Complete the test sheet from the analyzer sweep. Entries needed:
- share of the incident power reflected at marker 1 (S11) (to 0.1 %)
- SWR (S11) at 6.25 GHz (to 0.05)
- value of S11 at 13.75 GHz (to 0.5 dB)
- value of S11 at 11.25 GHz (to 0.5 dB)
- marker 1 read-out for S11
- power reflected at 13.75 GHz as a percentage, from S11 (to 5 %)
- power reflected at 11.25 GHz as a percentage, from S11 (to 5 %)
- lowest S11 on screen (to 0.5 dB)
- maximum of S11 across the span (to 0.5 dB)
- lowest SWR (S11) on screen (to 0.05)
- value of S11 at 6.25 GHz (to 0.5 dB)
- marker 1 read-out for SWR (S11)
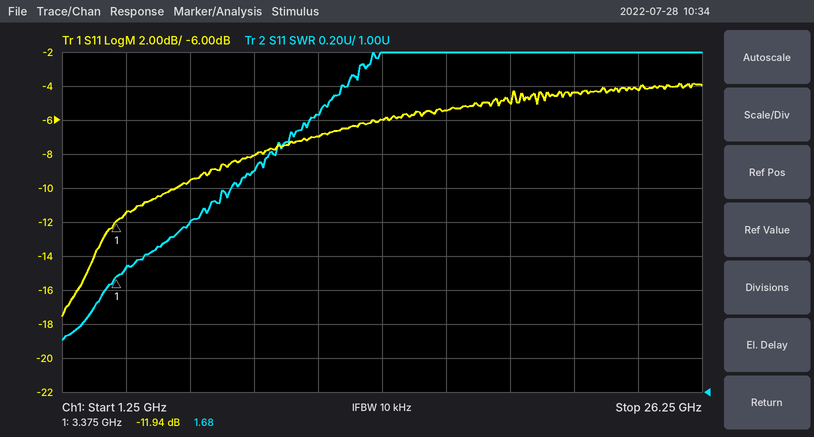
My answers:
6.4 %
2.00
-6.0 dB
-7.0 dB
-11.94 dB
25 %
20 %
-17.5 dB
-4.0 dB
1.30
-9.5 dB
1.68
